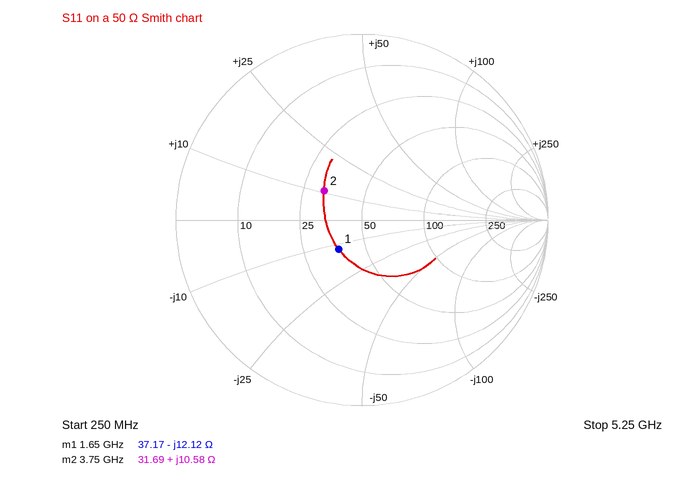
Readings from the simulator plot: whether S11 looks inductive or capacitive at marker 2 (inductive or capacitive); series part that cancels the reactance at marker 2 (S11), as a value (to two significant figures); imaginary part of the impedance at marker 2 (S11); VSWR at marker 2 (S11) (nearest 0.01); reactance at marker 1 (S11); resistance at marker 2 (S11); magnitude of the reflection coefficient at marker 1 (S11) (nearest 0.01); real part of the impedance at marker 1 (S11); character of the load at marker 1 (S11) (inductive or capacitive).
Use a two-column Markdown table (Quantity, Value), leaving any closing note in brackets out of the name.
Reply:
| Quantity | Value |
|---|---|
| whether S11 looks inductive or capacitive at marker 2 | inductive |
| series part that cancels the reactance at marker 2 (S11), as a value | 4.0 pF |
| imaginary part of the impedance at marker 2 | +10.58 Ω |
| VSWR at marker 2 (S11) | 1.69 |
| reactance at marker 1 | -12.12 Ω |
| resistance at marker 2 | 31.69 Ω |
| magnitude of the reflection coefficient at marker 1 (S11) | 0.20 |
| real part of the impedance at marker 1 | 37.17 Ω |
| character of the load at marker 1 (S11) | capacitive |
